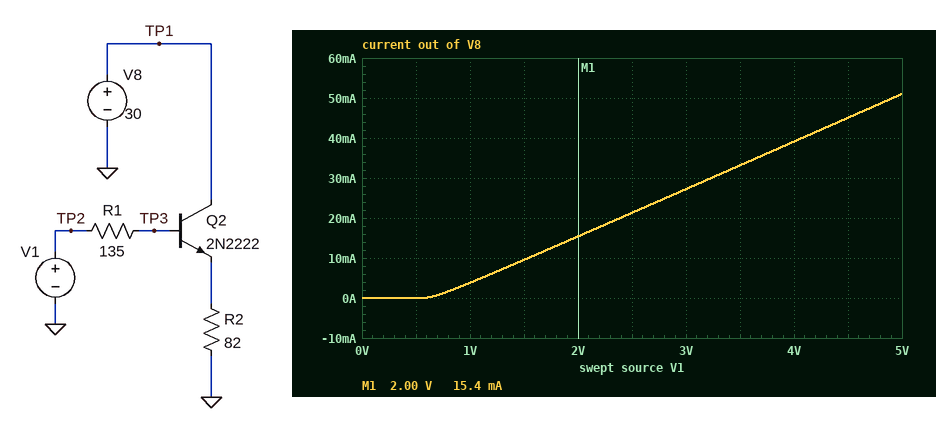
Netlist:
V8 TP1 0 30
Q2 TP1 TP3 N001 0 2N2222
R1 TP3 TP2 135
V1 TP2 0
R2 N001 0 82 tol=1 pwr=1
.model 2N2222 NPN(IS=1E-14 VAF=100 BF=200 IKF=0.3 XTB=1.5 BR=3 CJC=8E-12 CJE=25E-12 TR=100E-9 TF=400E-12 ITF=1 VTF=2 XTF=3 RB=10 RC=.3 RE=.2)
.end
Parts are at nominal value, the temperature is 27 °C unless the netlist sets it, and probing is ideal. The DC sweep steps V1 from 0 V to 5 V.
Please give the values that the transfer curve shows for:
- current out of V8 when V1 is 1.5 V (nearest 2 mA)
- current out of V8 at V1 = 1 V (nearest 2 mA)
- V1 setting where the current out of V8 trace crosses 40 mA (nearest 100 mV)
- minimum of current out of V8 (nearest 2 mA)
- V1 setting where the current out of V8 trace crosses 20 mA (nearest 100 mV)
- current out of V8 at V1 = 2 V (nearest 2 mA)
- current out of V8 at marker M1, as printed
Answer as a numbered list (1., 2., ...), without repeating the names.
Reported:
1. 10 mA
2. 4 mA
3. 4.1 V
4. 0 A
5. 2.4 V
6. 16 mA
7. 15.4 mA
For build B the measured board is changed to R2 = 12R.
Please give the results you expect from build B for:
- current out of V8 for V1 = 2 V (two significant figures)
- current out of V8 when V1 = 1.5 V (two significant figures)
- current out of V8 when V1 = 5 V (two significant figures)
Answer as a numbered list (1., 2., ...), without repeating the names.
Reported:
1. 95 mA
2. 58 mA
3. 310 mA
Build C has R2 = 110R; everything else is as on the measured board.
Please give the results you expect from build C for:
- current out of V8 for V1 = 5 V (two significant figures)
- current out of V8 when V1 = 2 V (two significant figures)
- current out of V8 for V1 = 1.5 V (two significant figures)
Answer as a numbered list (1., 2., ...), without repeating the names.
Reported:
1. 38 mA
2. 12 mA
3. 7.2 mA
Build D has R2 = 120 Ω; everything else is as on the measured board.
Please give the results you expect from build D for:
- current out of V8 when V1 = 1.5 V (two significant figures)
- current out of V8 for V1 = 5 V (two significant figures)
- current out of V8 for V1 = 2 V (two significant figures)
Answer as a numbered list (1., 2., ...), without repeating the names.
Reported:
1. 6.6 mA
2. 35 mA
3. 11 mA
